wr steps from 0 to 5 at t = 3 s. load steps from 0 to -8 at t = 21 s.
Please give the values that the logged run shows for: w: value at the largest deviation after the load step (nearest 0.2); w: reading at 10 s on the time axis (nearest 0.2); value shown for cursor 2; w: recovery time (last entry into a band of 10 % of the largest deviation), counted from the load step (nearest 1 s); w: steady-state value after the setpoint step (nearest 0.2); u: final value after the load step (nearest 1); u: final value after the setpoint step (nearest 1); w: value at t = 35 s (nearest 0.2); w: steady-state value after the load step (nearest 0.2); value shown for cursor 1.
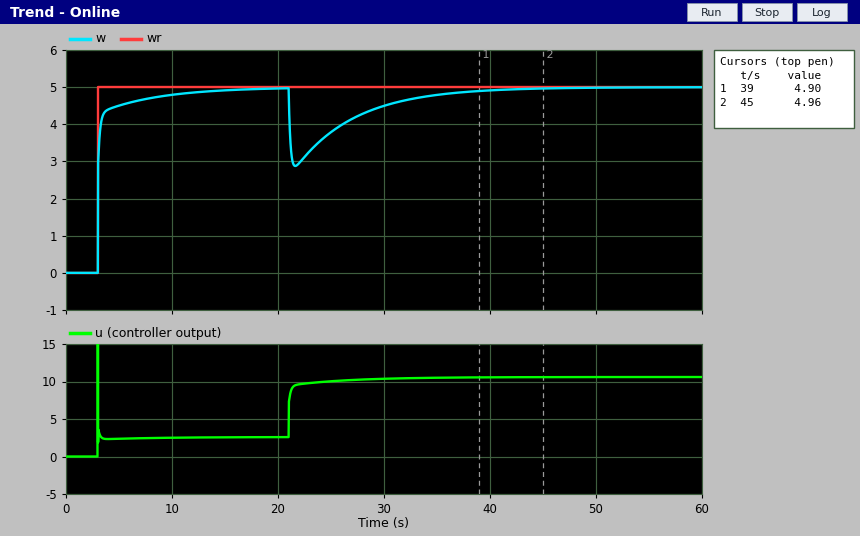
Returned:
2.8
4.8
4.96
14 s
5.0
11
3
4.8
5.0
4.90
